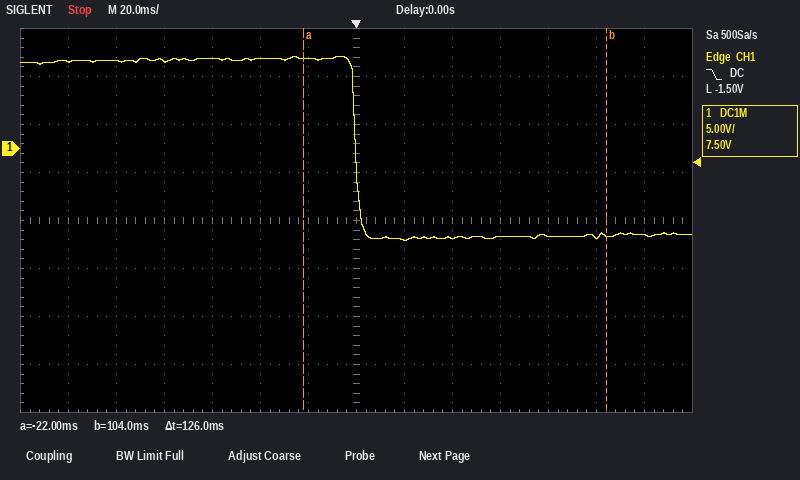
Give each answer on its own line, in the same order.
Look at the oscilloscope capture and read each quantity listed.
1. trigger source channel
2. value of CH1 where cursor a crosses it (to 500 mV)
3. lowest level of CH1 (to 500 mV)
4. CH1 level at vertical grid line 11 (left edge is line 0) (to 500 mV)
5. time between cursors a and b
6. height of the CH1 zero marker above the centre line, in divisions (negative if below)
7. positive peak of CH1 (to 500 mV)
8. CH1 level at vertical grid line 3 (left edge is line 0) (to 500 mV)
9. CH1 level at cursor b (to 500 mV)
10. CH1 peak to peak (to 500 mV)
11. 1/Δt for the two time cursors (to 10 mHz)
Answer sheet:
CH1
9.5 V
-9.5 V
-9.0 V
126 ms
+1.5 div
9.5 V
9.0 V
-9.0 V
19.0 V
7.94 Hz
